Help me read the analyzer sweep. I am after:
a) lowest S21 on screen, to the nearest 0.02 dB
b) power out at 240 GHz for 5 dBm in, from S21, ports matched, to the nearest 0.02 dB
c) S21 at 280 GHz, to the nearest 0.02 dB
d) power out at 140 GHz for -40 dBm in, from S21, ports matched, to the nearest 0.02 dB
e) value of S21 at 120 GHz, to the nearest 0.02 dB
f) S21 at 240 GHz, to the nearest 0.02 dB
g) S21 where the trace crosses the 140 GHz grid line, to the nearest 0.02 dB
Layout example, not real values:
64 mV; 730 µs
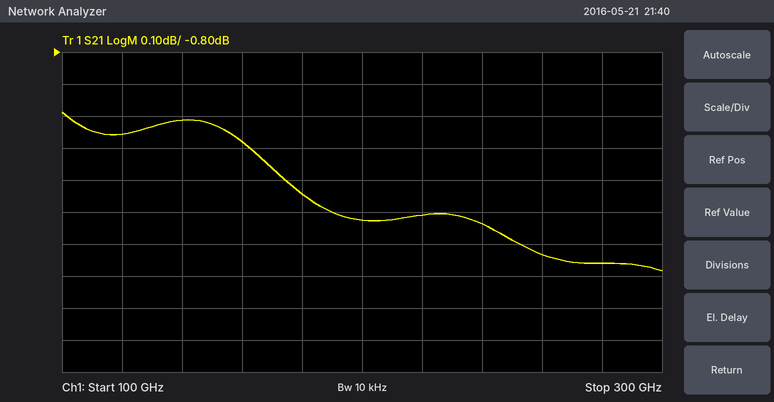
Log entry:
-1.48 dB; 3.66 dBm; -1.46 dB; -41.02 dBm; -1.06 dB; -1.34 dB; -1.02 dB
